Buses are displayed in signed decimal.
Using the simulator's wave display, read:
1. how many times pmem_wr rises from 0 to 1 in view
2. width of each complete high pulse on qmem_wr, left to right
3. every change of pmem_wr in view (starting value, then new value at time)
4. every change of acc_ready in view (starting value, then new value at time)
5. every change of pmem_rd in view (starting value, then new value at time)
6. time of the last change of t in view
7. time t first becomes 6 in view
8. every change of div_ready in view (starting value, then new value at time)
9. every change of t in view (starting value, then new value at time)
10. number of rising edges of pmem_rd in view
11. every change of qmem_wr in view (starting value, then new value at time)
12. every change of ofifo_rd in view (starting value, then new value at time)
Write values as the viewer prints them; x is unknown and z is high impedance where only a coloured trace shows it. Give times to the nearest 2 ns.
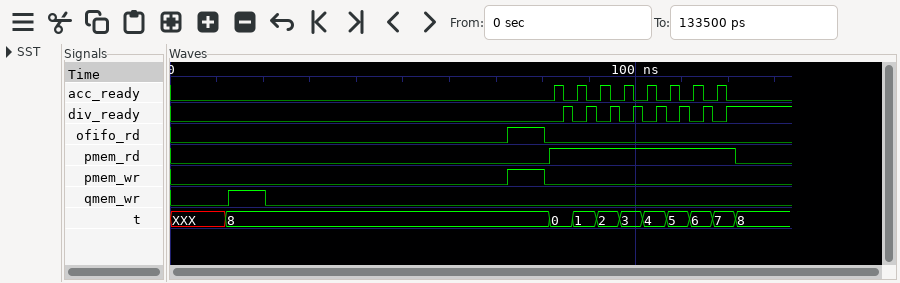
1
8 ns
0, 1 at 72 ns, 0 at 80 ns
0, 1 at 82 ns, 0 at 84 ns, 1 at 88 ns, 0 at 90 ns, 1 at 92 ns, 0 at 94 ns, 1 at 98 ns, 0 at 100 ns, 1 at 102 ns, 0 at 104 ns, 1 at 108 ns, 0 at 110 ns, 1 at 112 ns, 0 at 114 ns, 1 at 118 ns, 0 at 120 ns
0, 1 at 82 ns, 0 at 122 ns
122 ns
112 ns
0, 1 at 84 ns, 0 at 86 ns, 1 at 90 ns, 0 at 92 ns, 1 at 94 ns, 0 at 96 ns, 1 at 100 ns, 0 at 102 ns, 1 at 104 ns, 0 at 106 ns, 1 at 110 ns, 0 at 112 ns, 1 at 114 ns, 0 at 116 ns, 1 at 120 ns
XXX, 8 at 12 ns, 0 at 82 ns, 1 at 86 ns, 2 at 92 ns, 3 at 96 ns, 4 at 102 ns, 5 at 106 ns, 6 at 112 ns, 7 at 116 ns, 8 at 122 ns
1
0, 1 at 12 ns, 0 at 20 ns
0, 1 at 72 ns, 0 at 80 ns
